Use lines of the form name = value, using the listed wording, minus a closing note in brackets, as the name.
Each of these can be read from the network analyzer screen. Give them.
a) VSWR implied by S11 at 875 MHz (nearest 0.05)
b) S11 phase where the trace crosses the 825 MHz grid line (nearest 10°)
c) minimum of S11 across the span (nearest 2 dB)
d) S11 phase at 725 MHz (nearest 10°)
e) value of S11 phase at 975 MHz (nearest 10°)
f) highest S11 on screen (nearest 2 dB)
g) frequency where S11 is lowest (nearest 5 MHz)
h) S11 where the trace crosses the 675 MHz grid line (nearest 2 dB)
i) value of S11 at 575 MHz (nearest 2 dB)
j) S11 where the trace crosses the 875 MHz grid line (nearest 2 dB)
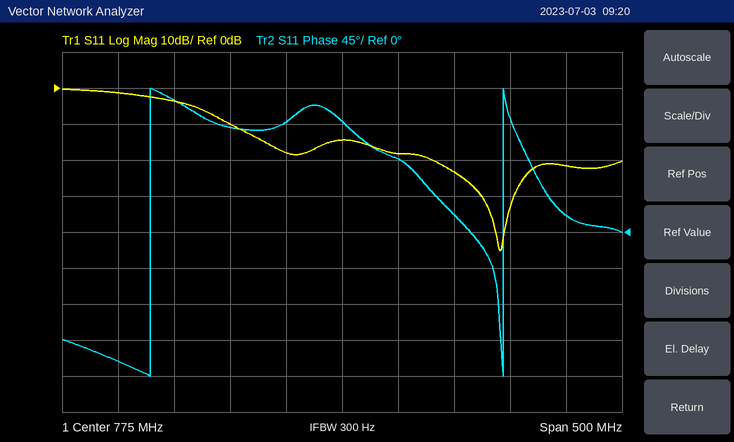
VSWR implied by S11 at 875 MHz = 1.15
S11 phase where the trace crosses the 825 MHz grid line = 90°
minimum of S11 across the span = -46 dB
S11 phase at 725 MHz = 140°
value of S11 phase at 975 MHz = 20°
highest S11 on screen = 0 dB
frequency where S11 is lowest = 915 MHz
S11 where the trace crosses the 675 MHz grid line = -10 dB
value of S11 at 575 MHz = -2 dB
S11 where the trace crosses the 875 MHz grid line = -24 dB
